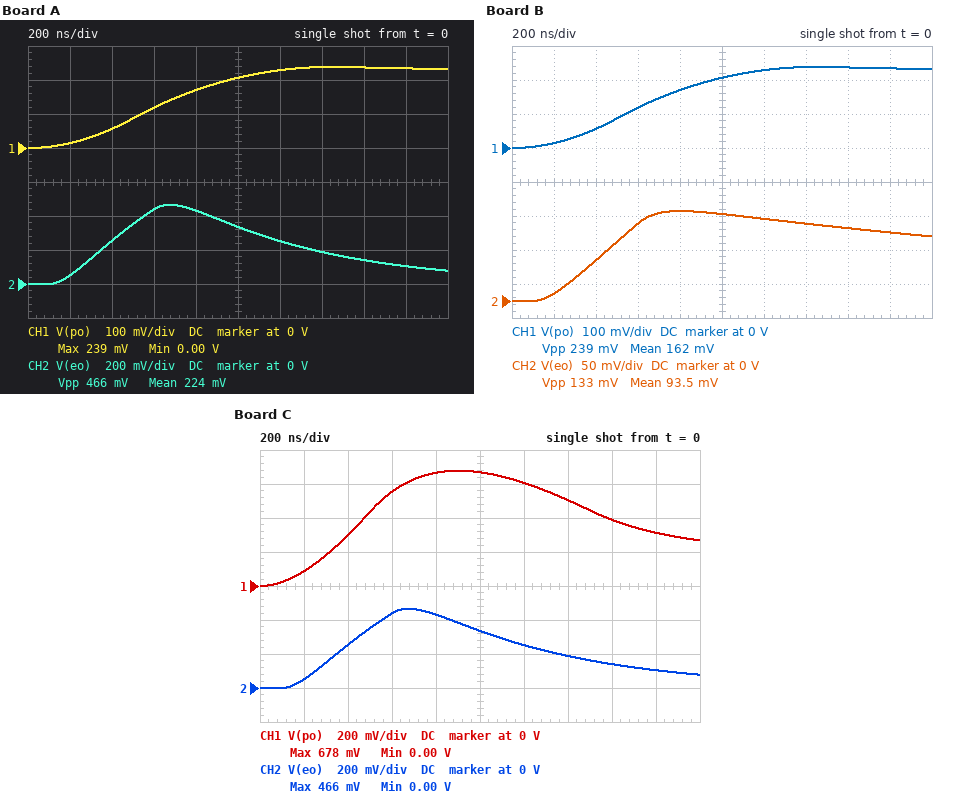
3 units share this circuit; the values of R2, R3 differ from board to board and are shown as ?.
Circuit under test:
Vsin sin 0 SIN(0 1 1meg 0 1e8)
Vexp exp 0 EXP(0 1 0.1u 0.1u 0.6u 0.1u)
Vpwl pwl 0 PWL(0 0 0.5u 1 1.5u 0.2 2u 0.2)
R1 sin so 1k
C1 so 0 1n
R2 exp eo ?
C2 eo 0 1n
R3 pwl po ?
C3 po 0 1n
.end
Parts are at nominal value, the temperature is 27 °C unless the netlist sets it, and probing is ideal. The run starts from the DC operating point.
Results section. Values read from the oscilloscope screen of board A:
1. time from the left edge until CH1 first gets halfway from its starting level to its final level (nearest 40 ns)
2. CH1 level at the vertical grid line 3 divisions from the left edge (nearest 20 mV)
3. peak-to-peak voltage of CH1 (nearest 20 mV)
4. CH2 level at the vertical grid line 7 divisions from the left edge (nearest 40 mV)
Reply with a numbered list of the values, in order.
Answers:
1. 600 ns
2. 120 mV
3. 240 mV
4. 200 mV
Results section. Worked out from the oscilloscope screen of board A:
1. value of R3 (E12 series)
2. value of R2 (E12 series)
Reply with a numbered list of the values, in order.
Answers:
1. 2.7 kΩ
2. 680 Ω
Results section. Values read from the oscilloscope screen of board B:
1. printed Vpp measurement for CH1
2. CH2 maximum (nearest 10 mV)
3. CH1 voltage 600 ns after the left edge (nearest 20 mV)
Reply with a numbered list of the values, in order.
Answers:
1. 239 mV
2. 130 mV
3. 120 mV
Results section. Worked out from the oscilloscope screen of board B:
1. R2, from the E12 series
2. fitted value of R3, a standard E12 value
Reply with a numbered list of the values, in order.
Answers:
1. 3.3 kΩ
2. 2.7 kΩ
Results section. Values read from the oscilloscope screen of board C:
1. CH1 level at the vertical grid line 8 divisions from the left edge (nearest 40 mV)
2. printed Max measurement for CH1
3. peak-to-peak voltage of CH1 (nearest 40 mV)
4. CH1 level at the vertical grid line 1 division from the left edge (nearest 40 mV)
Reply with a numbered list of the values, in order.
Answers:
1. 400 mV
2. 678 mV
3. 680 mV
4. 80 mV
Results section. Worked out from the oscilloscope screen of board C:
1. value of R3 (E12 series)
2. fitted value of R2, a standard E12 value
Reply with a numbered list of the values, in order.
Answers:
1. 390 Ω
2. 680 Ω
